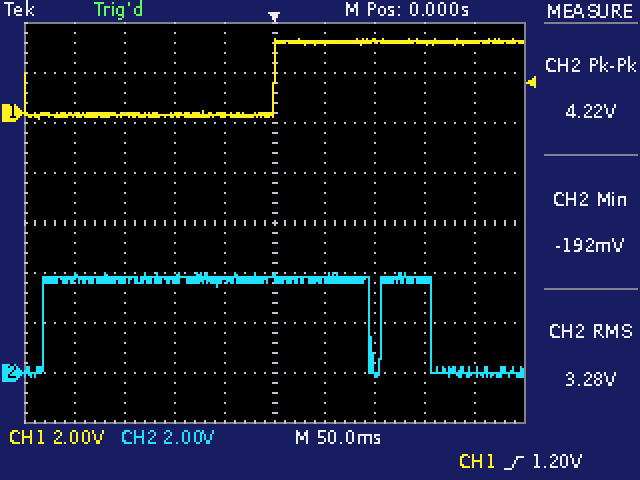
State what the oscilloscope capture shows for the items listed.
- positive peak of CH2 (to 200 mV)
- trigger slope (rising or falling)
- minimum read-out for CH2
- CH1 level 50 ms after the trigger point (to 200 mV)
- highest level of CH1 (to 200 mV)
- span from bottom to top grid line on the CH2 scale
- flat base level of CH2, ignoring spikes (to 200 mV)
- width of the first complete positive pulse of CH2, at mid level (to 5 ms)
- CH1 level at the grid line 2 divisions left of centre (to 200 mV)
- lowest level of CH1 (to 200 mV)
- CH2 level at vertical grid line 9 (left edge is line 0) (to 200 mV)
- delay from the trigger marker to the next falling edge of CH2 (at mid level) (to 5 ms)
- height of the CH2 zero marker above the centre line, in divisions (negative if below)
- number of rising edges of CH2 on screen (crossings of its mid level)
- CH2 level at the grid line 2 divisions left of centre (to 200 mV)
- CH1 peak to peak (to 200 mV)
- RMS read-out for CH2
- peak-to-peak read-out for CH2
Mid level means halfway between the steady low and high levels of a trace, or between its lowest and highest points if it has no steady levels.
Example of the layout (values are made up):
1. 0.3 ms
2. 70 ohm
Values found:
1. 4.0 V
2. rising
3. -192 mV
4. 2.8 V
5. 3.0 V
6. 16 V
7. 0.0 V
8. 325 ms
9. 0.0 V
10. -200 mV
11. 0.0 V
12. 95 ms
13. -3.0 div
14. 2
15. 3.8 V
16. 3.2 V
17. 3.28 V
18. 4.22 V
